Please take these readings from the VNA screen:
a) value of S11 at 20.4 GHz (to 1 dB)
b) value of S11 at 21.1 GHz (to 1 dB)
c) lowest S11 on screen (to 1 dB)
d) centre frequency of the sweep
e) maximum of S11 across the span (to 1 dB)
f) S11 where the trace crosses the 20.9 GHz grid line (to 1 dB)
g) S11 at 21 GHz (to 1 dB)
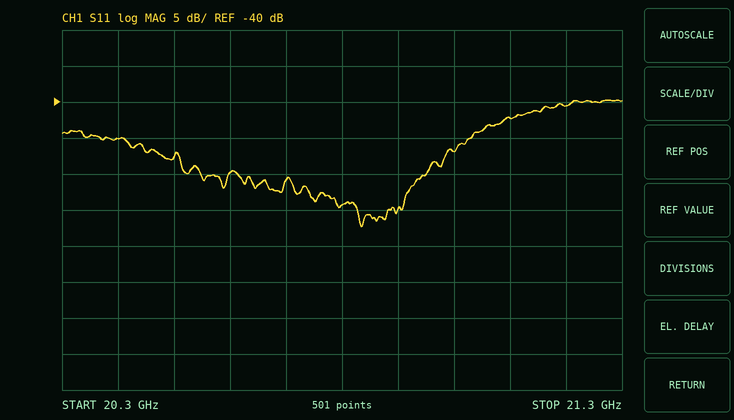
-45 dB
-42 dB
-57 dB
20.8 GHz
-40 dB
-55 dB
-47 dB
